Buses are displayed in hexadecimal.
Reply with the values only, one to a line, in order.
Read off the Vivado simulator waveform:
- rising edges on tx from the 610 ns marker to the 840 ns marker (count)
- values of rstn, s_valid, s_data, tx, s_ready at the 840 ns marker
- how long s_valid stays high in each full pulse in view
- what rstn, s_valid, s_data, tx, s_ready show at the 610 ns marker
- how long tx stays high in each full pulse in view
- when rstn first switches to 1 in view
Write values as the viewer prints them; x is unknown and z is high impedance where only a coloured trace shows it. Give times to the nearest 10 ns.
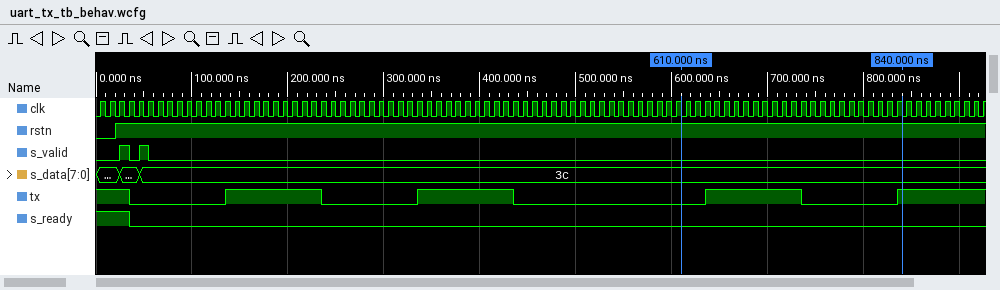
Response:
2
rstn=1, s_valid=0, s_data=3c, tx=1, s_ready=0
10 ns, 10 ns
rstn=1, s_valid=0, s_data=3c, tx=0, s_ready=0
100 ns, 100 ns, 100 ns
20 ns
